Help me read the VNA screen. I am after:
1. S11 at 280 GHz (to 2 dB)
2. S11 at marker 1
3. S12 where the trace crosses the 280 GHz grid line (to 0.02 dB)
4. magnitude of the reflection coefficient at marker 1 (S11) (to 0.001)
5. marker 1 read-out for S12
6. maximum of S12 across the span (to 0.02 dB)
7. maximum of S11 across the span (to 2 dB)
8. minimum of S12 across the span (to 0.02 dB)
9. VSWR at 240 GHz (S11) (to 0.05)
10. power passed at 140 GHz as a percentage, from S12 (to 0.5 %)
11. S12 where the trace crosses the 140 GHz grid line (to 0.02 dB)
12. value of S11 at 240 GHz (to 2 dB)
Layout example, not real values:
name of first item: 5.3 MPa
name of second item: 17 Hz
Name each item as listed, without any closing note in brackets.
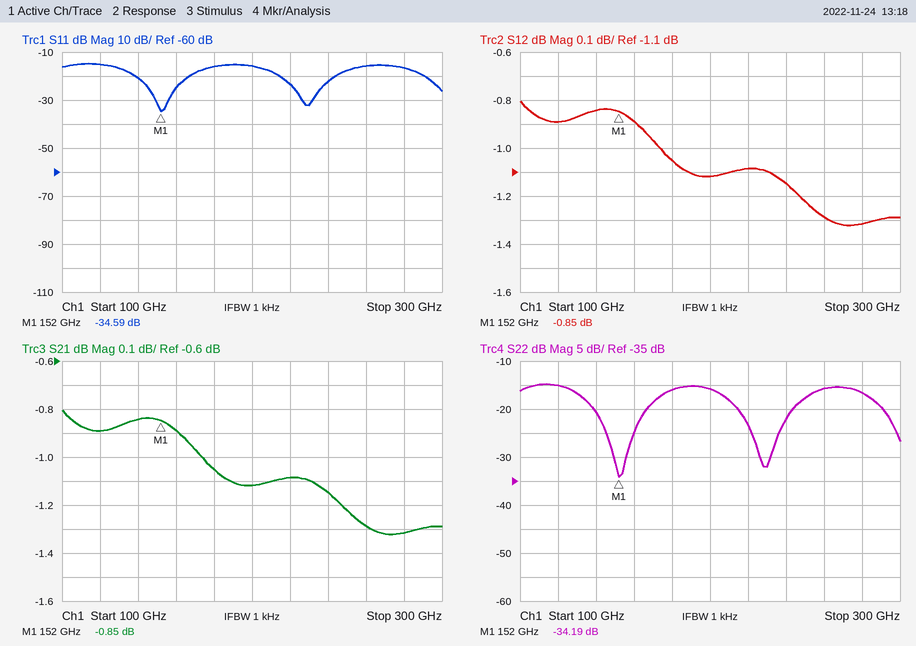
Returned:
S11 at 280 GHz: -16 dB
S11 at marker 1: -34.59 dB
S12 where the trace crosses the 280 GHz grid line: -1.32 dB
magnitude of the reflection coefficient at marker 1 (S11): 0.019
marker 1 read-out for S12: -0.85 dB
maximum of S12 across the span: -0.80 dB
maximum of S11 across the span: -14 dB
minimum of S12 across the span: -1.32 dB
VSWR at 240 GHz (S11): 1.15
power passed at 140 GHz as a percentage, from S12: 82.5 %
S12 where the trace crosses the 140 GHz grid line: -0.84 dB
value of S11 at 240 GHz: -22 dB
